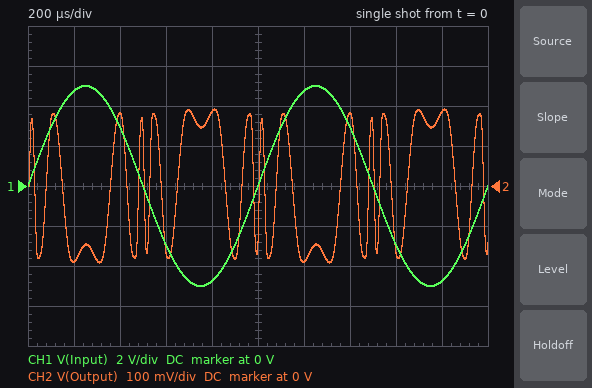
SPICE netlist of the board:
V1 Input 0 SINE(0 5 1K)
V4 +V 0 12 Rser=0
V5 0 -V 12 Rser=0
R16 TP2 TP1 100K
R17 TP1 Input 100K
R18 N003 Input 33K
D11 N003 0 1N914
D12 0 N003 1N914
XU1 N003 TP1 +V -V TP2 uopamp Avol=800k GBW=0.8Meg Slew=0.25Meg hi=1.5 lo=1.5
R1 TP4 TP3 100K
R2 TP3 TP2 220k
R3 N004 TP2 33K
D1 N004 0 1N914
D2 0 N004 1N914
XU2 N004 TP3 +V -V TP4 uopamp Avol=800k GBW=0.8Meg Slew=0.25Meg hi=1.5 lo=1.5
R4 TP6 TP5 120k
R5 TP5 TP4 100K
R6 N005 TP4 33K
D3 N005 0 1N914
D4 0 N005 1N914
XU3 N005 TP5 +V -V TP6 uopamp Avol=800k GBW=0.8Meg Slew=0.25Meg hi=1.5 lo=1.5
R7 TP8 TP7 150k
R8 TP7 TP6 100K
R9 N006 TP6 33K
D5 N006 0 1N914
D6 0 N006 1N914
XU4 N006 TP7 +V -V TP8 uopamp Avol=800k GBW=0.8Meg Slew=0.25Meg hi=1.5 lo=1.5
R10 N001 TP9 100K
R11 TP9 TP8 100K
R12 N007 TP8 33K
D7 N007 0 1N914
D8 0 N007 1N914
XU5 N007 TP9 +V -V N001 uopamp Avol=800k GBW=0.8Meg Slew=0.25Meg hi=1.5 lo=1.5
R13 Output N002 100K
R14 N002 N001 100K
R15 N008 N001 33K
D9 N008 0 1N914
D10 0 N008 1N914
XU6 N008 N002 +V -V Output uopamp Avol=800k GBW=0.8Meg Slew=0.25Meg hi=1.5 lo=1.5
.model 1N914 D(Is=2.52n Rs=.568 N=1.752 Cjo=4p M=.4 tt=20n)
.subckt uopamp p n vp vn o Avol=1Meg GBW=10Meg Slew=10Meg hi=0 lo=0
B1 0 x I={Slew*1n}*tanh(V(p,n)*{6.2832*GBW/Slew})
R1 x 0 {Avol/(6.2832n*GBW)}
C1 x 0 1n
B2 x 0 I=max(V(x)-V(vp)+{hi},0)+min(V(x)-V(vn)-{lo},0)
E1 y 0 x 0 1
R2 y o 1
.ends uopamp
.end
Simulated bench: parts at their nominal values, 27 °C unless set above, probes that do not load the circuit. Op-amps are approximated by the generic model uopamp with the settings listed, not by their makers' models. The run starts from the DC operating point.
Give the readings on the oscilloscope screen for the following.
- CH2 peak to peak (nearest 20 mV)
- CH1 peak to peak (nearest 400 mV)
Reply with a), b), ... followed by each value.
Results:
a) 380 mV
b) 10.0 V
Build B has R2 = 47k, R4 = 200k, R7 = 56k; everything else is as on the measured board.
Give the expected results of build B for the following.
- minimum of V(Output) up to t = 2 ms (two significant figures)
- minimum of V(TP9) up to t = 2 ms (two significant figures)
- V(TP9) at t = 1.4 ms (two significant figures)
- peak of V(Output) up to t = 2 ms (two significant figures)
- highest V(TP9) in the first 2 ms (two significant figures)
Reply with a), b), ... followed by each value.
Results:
a) -3.1 V
b) -500 mV
c) 430 mV
d) 3.1 V
e) 500 mV
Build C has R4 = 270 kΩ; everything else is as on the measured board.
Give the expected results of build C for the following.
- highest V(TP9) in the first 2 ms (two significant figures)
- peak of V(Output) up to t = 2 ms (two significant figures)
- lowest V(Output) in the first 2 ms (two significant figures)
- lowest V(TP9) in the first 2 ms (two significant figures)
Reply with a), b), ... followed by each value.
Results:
a) 410 mV
b) 240 mV
c) -240 mV
d) -410 mV
